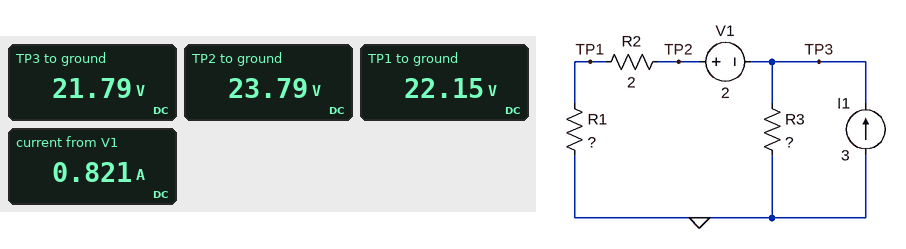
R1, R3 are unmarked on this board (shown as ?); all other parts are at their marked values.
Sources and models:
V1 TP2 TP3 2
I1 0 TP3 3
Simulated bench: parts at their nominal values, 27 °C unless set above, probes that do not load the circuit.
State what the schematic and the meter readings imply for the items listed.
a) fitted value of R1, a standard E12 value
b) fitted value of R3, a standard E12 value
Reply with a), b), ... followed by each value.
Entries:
a) 27 Ω
b) 10 Ω
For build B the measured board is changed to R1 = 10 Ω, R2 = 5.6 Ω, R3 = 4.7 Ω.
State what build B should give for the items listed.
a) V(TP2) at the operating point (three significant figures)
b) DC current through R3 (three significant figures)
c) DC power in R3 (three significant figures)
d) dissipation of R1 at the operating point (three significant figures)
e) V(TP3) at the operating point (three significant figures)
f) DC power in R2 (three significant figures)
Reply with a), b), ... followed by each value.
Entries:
a) 12.4 V
b) 2.21 A
c) 22.9 W
d) 6.29 W
e) 10.4 V
f) 3.52 W
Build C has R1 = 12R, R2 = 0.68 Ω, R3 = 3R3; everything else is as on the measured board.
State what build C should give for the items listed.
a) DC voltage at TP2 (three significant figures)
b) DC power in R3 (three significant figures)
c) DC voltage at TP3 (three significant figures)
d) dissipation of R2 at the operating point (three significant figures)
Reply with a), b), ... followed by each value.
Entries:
a) 9.44 V
b) 16.8 W
c) 7.44 V
d) 377 mW
